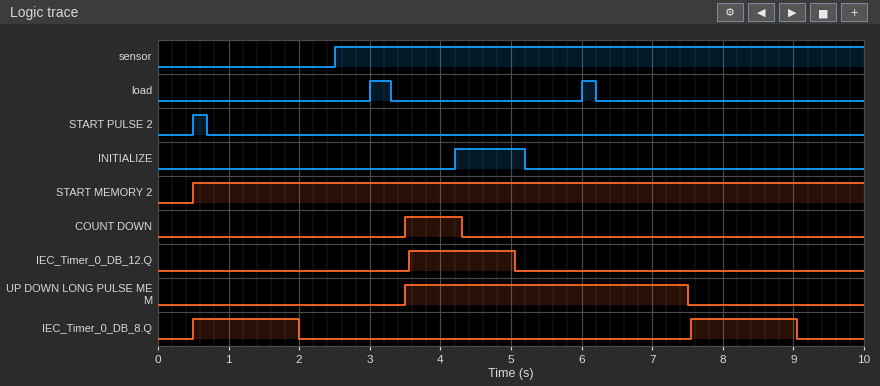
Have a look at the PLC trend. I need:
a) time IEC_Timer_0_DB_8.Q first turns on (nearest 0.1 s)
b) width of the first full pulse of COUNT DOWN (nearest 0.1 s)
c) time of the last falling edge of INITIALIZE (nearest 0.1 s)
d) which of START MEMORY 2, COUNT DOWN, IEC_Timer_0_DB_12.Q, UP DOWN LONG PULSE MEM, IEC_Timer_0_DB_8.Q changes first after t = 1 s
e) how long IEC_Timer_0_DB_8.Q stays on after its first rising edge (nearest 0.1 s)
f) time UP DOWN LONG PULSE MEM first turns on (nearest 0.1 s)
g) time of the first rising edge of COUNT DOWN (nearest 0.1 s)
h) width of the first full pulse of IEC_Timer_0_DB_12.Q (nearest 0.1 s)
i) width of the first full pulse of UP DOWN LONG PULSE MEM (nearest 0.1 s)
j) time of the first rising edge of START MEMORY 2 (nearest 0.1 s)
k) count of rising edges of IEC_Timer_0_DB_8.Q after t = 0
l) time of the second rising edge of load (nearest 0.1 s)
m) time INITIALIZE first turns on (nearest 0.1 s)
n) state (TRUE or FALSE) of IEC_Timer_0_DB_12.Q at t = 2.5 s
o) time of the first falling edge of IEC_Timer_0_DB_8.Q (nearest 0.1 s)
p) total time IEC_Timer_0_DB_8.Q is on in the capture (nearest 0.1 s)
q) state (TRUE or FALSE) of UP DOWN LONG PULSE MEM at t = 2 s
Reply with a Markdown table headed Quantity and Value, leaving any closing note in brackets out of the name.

| Quantity | Value |
|---|---|
| time IEC_Timer_0_DB_8.Q first turns on | 0.5 s |
| width of the first full pulse of COUNT DOWN | 0.8 s |
| time of the last falling edge of INITIALIZE | 5.2 s |
| which of START MEMORY 2, COUNT DOWN, IEC_Timer_0_DB_12.Q, UP DOWN LONG PULSE MEM, IEC_Timer_0_DB_8.Q changes first after t = 1 s | IEC_Timer_0_DB_8.Q |
| how long IEC_Timer_0_DB_8.Q stays on after its first rising edge | 1.5 s |
| time UP DOWN LONG PULSE MEM first turns on | 3.5 s |
| time of the first rising edge of COUNT DOWN | 3.5 s |
| width of the first full pulse of IEC_Timer_0_DB_12.Q | 1.5 s |
| width of the first full pulse of UP DOWN LONG PULSE MEM | 4.0 s |
| time of the first rising edge of START MEMORY 2 | 0.5 s |
| count of rising edges of IEC_Timer_0_DB_8.Q after t = 0 | 2 |
| time of the second rising edge of load | 6.0 s |
| time INITIALIZE first turns on | 4.2 s |
| state (TRUE or FALSE) of IEC_Timer_0_DB_12.Q at t = 2.5 s | FALSE |
| time of the first falling edge of IEC_Timer_0_DB_8.Q | 2.0 s |
| total time IEC_Timer_0_DB_8.Q is on in the capture | 3.0 s |
| state (TRUE or FALSE) of UP DOWN LONG PULSE MEM at t = 2 s | FALSE |
